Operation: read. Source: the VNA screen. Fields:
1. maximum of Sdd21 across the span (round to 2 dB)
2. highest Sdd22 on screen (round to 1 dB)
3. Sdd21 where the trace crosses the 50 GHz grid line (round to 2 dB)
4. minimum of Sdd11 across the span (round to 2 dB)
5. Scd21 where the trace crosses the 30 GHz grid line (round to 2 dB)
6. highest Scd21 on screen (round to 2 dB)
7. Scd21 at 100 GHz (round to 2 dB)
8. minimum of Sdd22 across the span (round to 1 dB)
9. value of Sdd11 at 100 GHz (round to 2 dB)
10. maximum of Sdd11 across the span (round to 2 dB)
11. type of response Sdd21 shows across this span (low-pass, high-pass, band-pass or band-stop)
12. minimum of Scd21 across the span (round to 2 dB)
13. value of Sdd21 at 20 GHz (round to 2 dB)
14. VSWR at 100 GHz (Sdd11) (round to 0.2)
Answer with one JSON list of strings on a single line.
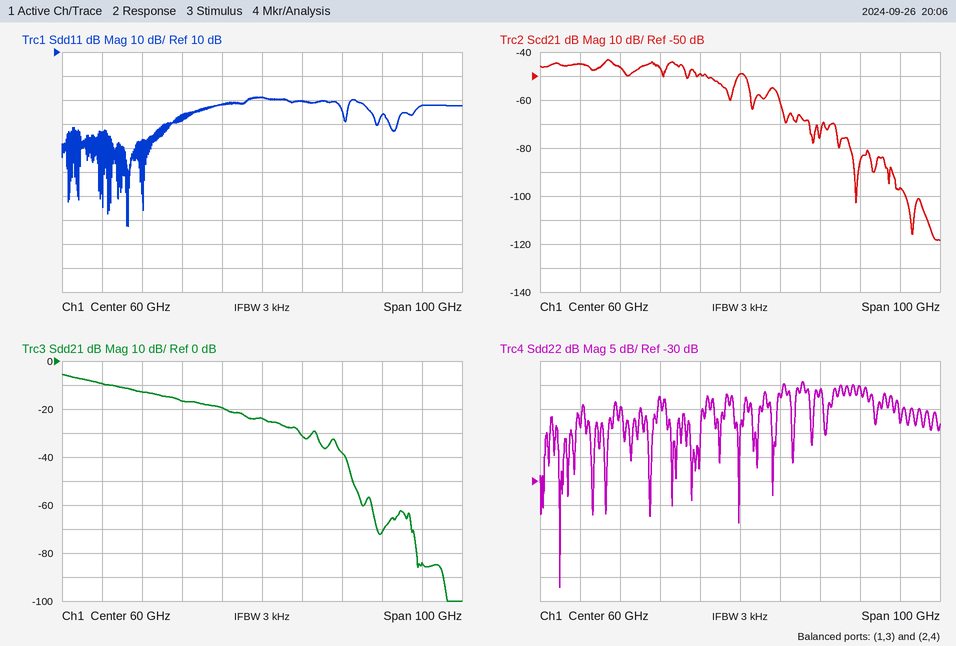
["-6 dB", "-9 dB", "-20 dB", "-62 dB", "-46 dB", "-44 dB", "-96 dB", "-52 dB", "-12 dB", "-8 dB", "low-pass", "-118 dB", "-10 dB", "1.6"]
